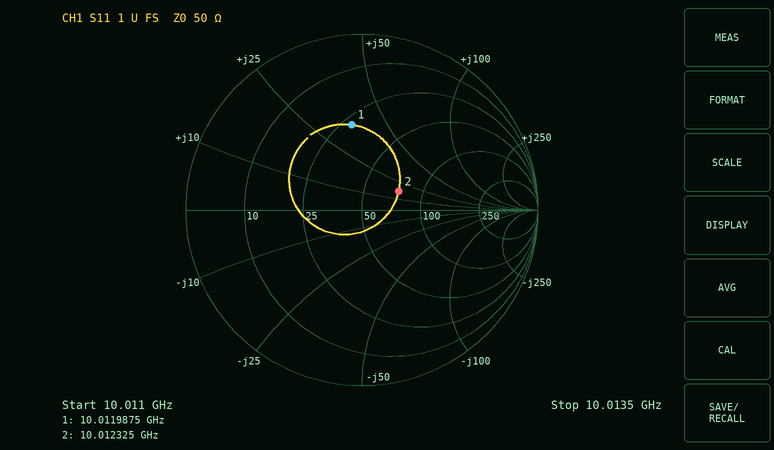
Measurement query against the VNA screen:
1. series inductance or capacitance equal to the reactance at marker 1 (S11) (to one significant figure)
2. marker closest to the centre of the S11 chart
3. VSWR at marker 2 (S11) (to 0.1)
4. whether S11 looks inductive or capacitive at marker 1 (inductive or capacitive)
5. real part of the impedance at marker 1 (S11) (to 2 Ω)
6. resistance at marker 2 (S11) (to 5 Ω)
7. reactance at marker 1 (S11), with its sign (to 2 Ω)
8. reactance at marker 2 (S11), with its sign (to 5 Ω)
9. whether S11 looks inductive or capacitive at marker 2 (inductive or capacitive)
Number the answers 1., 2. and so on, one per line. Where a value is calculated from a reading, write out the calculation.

1. L = 36 Ω/(2π × 10.0119875 GHz) ≈ 572 pH, so 600 pH to one significant figure
2. marker 2
3. 1.6
4. inductive
5. 28 Ω
6. 75 Ω
7. +36 Ω
8. +15 Ω
9. inductive
